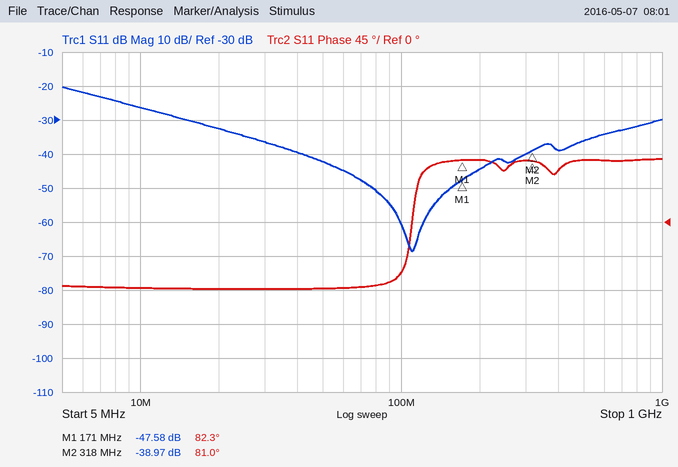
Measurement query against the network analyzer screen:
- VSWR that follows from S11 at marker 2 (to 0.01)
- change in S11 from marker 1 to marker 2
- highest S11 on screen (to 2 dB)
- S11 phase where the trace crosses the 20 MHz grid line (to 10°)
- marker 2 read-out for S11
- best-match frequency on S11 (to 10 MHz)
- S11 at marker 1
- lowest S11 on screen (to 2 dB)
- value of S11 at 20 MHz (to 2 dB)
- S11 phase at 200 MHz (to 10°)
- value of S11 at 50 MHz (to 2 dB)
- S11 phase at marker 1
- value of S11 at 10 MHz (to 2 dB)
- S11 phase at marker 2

1.02
8.61 dB
-20 dB
-90°
-38.97 dB
110 MHz
-47.58 dB
-68 dB
-32 dB
80°
-42 dB
82.3°
-26 dB
81.0°
